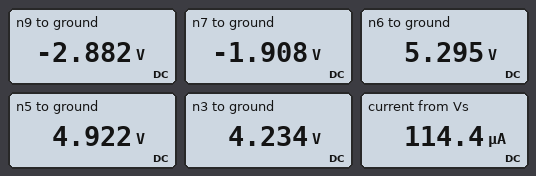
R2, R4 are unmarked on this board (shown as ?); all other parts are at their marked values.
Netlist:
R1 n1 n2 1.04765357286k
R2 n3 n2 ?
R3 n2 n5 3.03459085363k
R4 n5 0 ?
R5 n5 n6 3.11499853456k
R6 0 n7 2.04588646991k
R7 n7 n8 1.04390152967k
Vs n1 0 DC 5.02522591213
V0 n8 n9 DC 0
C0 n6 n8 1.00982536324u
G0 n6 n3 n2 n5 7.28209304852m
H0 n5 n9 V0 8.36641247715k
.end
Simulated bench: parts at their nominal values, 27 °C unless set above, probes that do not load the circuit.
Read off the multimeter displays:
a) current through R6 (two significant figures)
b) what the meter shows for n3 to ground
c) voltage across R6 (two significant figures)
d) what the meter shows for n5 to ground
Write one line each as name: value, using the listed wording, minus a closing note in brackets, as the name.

current through R6: 930 µA
what the meter shows for n3 to ground: 4.234 V
voltage across R6: 1.9 V
what the meter shows for n5 to ground: 4.922 V
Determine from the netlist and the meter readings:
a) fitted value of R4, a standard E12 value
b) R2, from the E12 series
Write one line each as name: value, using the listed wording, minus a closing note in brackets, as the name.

fitted value of R4, a standard E12 value: 4.7 kΩ
R2, from the E12 series: 5.6 kΩ
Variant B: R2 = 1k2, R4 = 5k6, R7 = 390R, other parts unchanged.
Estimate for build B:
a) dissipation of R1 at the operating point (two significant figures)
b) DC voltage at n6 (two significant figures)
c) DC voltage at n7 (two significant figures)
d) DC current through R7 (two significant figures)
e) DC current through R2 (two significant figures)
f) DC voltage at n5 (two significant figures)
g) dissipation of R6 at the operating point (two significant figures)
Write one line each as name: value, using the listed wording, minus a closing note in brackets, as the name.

dissipation of R1 at the operating point: 2.6 µW
DC voltage at n6: 5.1 V
DC voltage at n7: -1.7 V
DC current through R7: 840 µA
DC current through R2: 52 µA
DC voltage at n5: 5.0 V
dissipation of R6 at the operating point: 1.4 mW
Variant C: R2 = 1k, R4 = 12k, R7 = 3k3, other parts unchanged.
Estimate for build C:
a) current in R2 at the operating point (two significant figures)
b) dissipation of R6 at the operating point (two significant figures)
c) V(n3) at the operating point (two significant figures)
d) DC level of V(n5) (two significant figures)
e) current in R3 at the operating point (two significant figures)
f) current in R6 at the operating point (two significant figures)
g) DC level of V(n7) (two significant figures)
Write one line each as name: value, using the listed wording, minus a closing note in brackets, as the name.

current in R2 at the operating point: 1.7 mA
dissipation of R6 at the operating point: 9.4 mW
V(n3) at the operating point: 8.4 V
DC level of V(n5): 6.5 V
current in R3 at the operating point: 76 µA
current in R6 at the operating point: 2.1 mA
DC level of V(n7): -4.4 V
